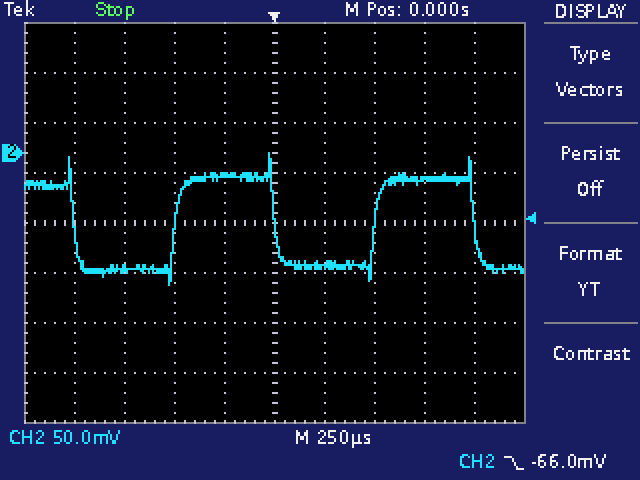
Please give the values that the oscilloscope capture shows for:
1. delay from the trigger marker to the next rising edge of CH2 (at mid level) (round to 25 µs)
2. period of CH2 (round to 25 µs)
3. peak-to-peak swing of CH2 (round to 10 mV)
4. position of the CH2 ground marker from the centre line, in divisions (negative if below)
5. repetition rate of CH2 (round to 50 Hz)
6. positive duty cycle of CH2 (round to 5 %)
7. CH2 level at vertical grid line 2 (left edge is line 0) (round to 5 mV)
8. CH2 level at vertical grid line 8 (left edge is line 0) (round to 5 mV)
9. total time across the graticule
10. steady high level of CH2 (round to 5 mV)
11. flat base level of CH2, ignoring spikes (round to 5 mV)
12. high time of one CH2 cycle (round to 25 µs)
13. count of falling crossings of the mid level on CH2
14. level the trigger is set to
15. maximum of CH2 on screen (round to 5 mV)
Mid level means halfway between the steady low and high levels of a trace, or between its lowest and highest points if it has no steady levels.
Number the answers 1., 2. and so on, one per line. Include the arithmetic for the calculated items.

1. 500 µs
2. 1.000 ms
3. 130 mV
4. +1.4 div
5. 1 / 1.000 ms ≈ 1.00 kHz
6. 500 µs / 1.000 ms ≈ 50 %
7. -115 mV
8. -25 mV
9. 2.5 ms
10. -25 mV
11. -115 mV
12. 500 µs
13. 3
14. -66.0 mV
15. 0 mV
